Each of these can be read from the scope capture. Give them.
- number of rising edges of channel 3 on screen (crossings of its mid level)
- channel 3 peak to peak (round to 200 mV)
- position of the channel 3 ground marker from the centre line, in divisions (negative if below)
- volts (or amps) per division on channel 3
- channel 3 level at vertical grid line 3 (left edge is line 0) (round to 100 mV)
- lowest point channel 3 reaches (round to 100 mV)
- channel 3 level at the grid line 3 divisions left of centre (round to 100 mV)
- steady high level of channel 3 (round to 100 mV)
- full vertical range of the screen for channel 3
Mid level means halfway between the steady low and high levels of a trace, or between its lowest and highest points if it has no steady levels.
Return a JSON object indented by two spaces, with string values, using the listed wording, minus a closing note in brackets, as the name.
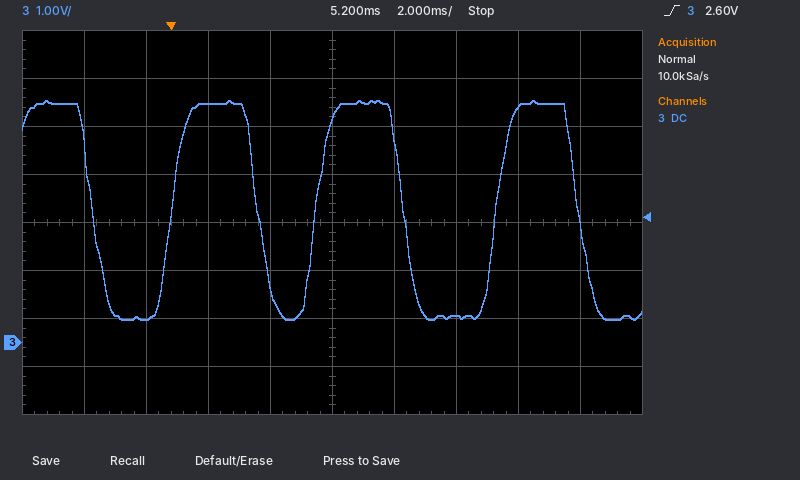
{
  "number of rising edges of channel 3 on screen": "3",
  "channel 3 peak to peak": "4.6 V",
  "position of the channel 3 ground marker from the centre line, in divisions": "-2.5 div",
  "volts (or amps) per division on channel 3": "1 V",
  "channel 3 level at vertical grid line 3 (left edge is line 0)": "5.0 V",
  "lowest point channel 3 reaches": "500 mV",
  "channel 3 level at the grid line 3 divisions left of centre": "500 mV",
  "steady high level of channel 3": "5.0 V",
  "full vertical range of the screen for channel 3": "8 V"
}
